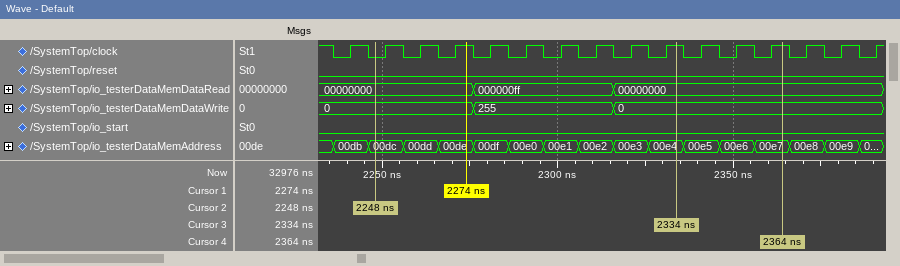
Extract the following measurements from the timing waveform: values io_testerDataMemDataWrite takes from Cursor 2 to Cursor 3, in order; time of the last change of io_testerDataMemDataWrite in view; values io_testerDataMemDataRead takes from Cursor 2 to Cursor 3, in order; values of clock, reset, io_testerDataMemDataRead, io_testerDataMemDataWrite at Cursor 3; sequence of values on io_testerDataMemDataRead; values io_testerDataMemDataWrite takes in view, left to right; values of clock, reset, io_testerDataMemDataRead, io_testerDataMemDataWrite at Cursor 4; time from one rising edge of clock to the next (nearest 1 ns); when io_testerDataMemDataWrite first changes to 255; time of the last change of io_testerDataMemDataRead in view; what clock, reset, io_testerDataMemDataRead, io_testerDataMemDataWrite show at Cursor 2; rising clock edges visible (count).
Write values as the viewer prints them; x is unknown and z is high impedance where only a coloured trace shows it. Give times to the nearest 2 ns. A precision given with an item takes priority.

0, 255, 0
2316 ns
00000000, 000000ff, 00000000
clock=1, reset=0, io_testerDataMemDataRead=00000000, io_testerDataMemDataWrite=0
00000000, 000000ff, 00000000
0, 255, 0
clock=1, reset=0, io_testerDataMemDataRead=00000000, io_testerDataMemDataWrite=0
10 ns
2276 ns
2316 ns
clock=0, reset=0, io_testerDataMemDataRead=00000000, io_testerDataMemDataWrite=0
16
